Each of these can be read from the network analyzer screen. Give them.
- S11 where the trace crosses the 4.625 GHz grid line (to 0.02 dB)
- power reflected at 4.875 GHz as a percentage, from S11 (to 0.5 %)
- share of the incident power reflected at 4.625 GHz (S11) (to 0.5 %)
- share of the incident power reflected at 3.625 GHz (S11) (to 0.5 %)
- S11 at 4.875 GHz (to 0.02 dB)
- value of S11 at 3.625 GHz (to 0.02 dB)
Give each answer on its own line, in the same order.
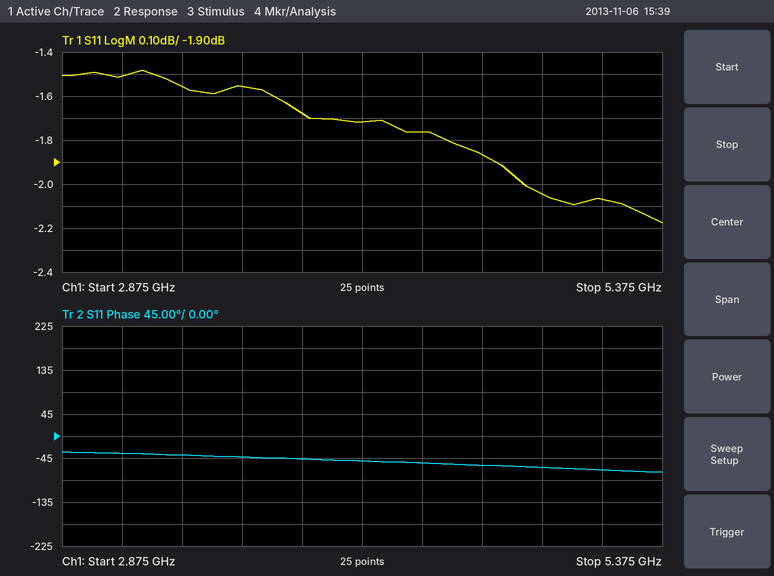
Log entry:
-1.86 dB
62.5 %
65.0 %
70.0 %
-2.04 dB
-1.56 dB
